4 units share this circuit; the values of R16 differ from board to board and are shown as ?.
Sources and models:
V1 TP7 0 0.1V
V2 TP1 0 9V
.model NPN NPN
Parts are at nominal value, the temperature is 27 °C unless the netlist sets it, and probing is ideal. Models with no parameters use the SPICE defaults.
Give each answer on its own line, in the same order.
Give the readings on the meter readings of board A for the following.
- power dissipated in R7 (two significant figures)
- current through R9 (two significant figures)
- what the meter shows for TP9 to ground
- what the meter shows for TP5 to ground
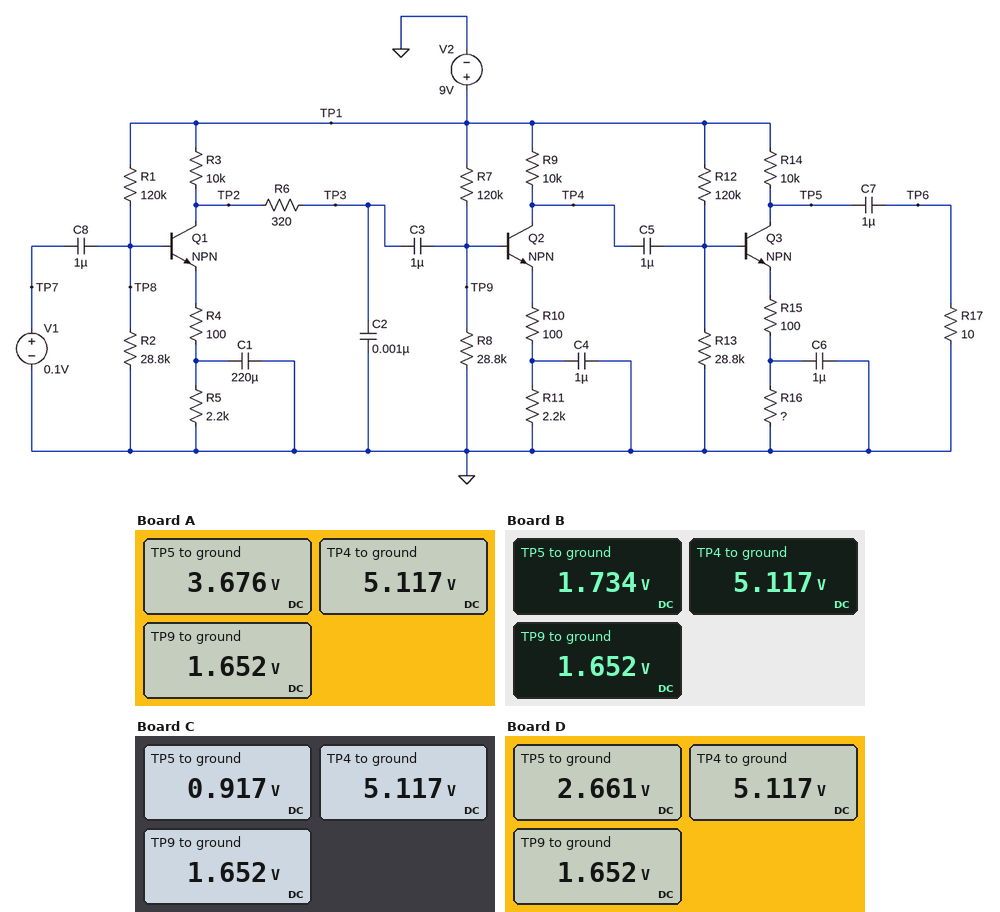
450 µW
390 µA
1.652 V
3.676 V
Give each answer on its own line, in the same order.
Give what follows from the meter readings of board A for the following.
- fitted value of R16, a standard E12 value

1.5 kΩ
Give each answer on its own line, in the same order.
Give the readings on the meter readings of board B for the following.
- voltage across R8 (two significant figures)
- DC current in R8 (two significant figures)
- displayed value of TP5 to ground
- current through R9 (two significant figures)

1.7 V
57 µA
1.734 V
390 µA
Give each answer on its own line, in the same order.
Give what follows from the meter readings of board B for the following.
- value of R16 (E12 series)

1 kΩ
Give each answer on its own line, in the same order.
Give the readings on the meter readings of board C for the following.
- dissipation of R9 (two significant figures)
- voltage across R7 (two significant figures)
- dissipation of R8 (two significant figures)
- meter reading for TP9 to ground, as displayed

1.5 mW
7.3 V
95 µW
1.652 V
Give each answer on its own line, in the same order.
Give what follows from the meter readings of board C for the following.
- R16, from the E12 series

820 Ω
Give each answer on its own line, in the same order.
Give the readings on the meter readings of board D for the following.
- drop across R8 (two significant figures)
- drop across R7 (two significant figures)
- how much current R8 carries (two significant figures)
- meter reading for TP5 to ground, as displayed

1.7 V
7.3 V
57 µA
2.661 V
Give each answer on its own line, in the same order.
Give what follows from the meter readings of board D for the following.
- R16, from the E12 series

1.2 kΩ
